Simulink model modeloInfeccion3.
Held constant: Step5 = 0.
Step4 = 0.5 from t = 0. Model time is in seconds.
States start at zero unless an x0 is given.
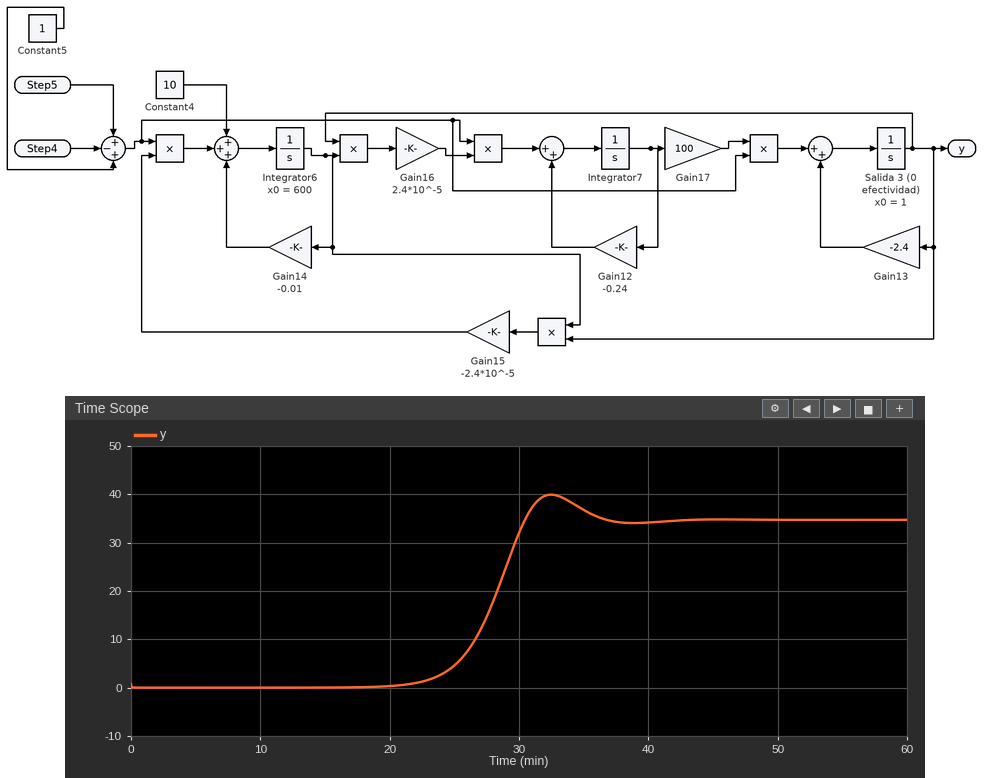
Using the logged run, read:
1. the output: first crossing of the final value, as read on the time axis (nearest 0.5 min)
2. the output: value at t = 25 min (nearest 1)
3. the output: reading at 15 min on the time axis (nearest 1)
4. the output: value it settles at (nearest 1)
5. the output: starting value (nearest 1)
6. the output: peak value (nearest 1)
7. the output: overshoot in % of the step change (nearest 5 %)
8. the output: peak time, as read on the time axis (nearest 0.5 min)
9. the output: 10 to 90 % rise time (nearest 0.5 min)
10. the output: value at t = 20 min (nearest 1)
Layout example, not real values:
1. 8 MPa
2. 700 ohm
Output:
1. 30.5 min
2. 5
3. 0
4. 35
5. 1
6. 40
7. 15 %
8. 32.5 min
9. 5.0 min
10. 0
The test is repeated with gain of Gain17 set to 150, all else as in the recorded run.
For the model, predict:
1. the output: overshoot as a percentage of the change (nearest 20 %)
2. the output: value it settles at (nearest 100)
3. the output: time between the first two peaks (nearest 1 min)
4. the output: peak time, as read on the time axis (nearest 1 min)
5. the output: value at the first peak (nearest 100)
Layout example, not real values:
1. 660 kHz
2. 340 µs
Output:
1. 260 %
2. 500
3. 3 min
4. 3 min
5. 1700
